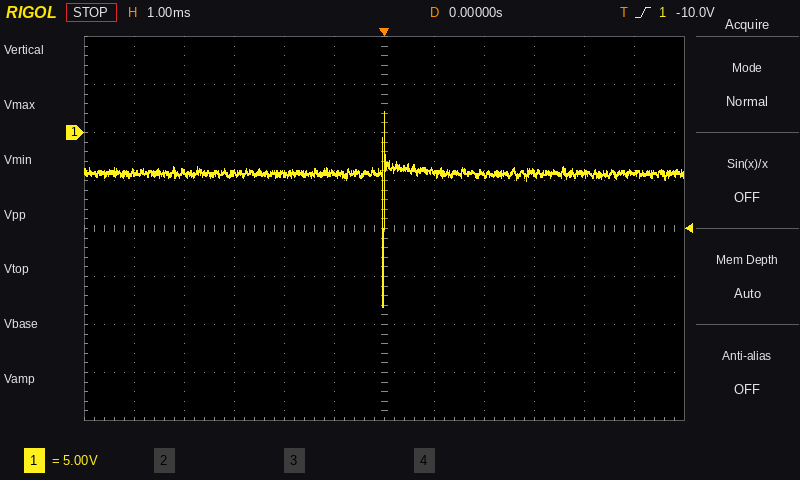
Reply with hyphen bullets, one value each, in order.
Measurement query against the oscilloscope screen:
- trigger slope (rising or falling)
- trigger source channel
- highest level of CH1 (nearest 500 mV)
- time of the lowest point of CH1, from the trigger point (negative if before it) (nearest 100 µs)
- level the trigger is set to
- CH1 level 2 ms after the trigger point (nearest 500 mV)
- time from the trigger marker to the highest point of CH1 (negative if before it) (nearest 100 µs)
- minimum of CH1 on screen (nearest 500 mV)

- rising
- CH1
- 2.0 V
- 0.0 ms
- -10.0 V
- -4.5 V
- 0.0 ms
- -18.0 V
